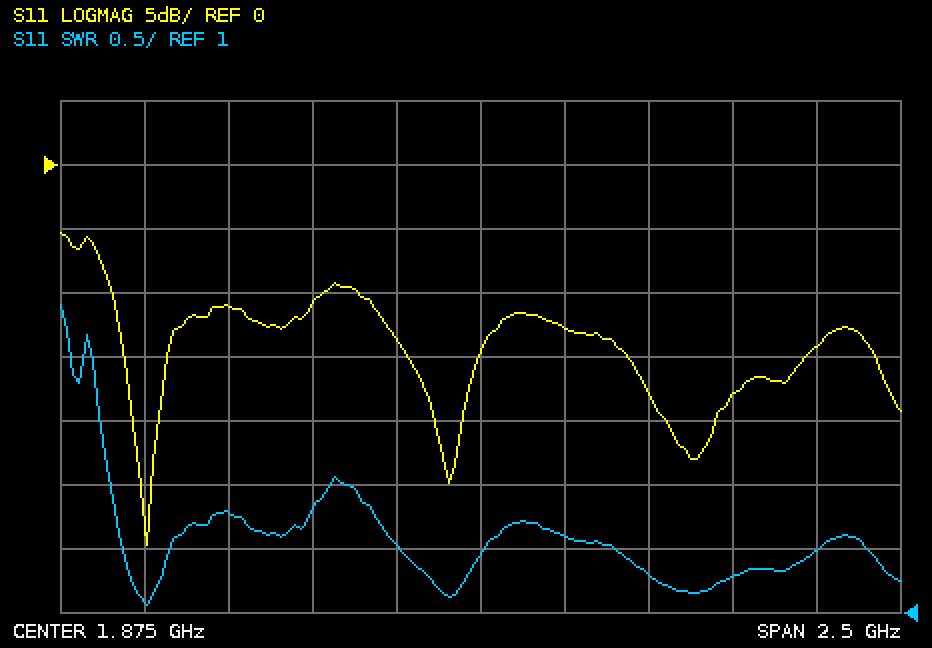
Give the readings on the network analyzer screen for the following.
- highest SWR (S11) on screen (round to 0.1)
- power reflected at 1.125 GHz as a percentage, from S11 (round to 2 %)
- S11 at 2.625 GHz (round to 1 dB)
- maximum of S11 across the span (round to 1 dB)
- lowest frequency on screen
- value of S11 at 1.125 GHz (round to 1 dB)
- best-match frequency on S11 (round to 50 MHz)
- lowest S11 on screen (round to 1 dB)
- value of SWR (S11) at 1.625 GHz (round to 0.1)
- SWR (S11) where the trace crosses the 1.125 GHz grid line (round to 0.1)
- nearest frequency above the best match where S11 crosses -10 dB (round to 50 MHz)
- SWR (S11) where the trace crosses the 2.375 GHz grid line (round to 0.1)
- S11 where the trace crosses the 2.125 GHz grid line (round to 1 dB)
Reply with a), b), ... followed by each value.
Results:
a) 3.4
b) 8 %
c) -18 dB
d) -5 dB
e) 625 MHz
f) -11 dB
g) 900 MHz
h) -30 dB
i) 1.5
j) 1.8
k) 1.40 GHz
l) 1.3
m) -13 dB
